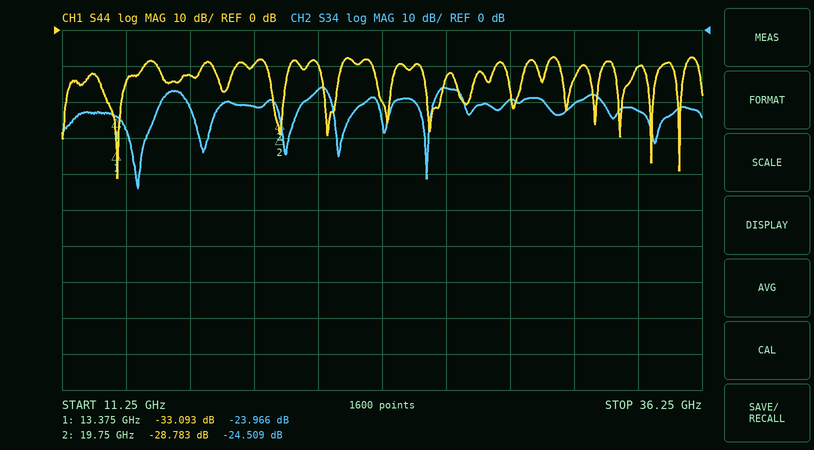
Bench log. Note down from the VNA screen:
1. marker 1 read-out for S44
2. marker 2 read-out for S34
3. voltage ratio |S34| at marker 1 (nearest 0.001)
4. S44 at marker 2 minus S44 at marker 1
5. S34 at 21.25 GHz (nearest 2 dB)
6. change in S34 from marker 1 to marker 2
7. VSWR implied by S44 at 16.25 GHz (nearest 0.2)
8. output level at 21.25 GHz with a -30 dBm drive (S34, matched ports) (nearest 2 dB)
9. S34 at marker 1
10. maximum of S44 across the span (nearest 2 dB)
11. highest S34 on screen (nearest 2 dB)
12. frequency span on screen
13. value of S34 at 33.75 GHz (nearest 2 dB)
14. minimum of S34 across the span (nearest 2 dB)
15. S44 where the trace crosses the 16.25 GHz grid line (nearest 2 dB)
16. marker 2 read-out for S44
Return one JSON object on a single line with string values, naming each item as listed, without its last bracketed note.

{"marker 1 read-out for S44": "-33.093 dB", "marker 2 read-out for S34": "-24.509 dB", "voltage ratio |S34| at marker 1": "0.063", "S44 at marker 2 minus S44 at marker 1": "4.310 dB", "S34 at 21.25 GHz": "-16 dB", "change in S34 from marker 1 to marker 2": "-0.543 dB", "VSWR implied by S44 at 16.25 GHz": "1.6", "output level at 21.25 GHz with a -30 dBm drive (S34, matched ports)": "-46 dBm", "S34 at marker 1": "-23.966 dB", "maximum of S44 across the span": "-8 dB", "highest S34 on screen": "-16 dB", "frequency span on screen": "25 GHz", "value of S34 at 33.75 GHz": "-22 dB", "minimum of S34 across the span": "-44 dB", "S44 where the trace crosses the 16.25 GHz grid line": "-12 dB", "marker 2 read-out for S44": "-28.783 dB"}
